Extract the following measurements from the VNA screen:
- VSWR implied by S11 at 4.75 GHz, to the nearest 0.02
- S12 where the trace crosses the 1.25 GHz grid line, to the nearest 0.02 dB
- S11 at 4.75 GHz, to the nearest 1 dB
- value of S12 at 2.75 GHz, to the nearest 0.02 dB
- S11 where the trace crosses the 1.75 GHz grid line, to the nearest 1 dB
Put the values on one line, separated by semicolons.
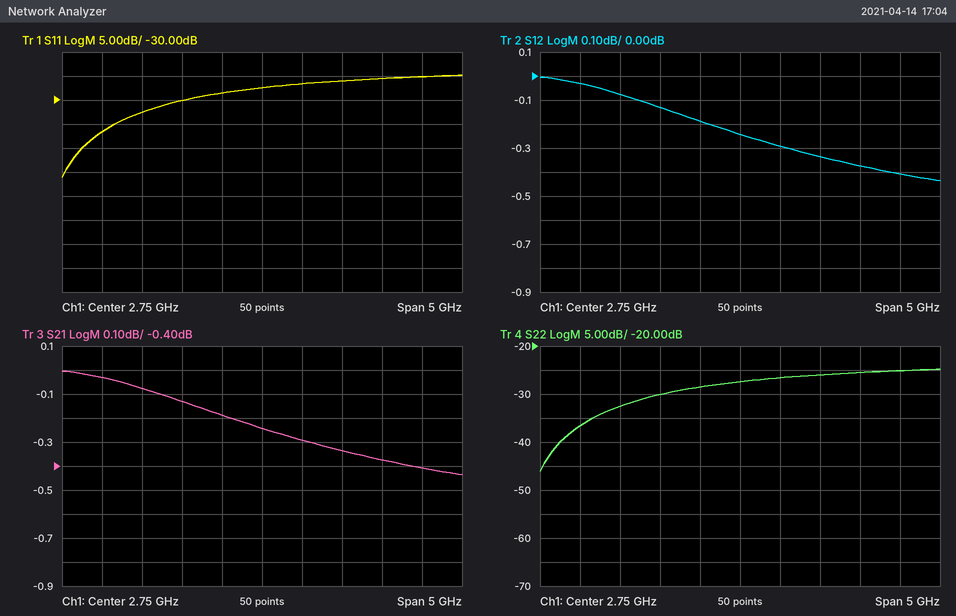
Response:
1.12; -0.08 dB; -25 dB; -0.24 dB; -30 dB
